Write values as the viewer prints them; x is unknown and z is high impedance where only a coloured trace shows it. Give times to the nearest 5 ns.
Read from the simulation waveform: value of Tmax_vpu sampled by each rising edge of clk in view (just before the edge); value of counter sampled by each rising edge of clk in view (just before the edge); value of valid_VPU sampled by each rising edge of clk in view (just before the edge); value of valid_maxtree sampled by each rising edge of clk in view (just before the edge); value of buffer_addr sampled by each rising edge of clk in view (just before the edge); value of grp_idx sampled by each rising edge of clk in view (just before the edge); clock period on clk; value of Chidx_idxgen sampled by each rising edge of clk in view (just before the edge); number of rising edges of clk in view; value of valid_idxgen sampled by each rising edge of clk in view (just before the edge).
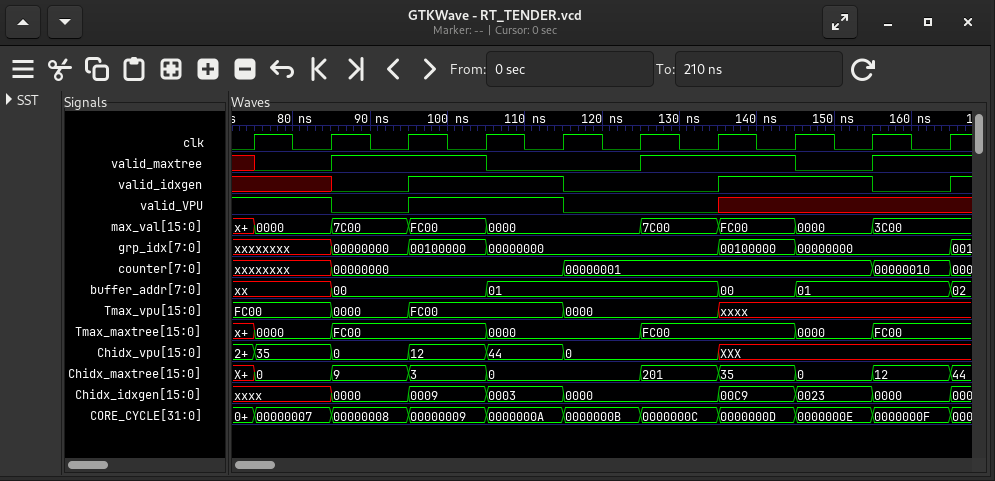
FC00, FC00, 0000, FC00, FC00, 0000, 0000, xxxx, xxxx, xxxx
xxxxxxxx, xxxxxxxx, 00000000, 00000000, 00000000, 00000001, 00000001, 00000001, 00000001, 00000010
1 1 0 1 1 0 0 x x x
x 0 1 1 0 0 1 1 0 1
xx, xx, 00, 00, 01, 01, 01, 00, 01, 01
xxxxxxxx, xxxxxxxx, 00000000, 00100000, 00000000, 00000000, 00000000, 00100000, 00000000, 00000000
10 ns
xxxx, xxxx, 0000, 0009, 0003, 0000, 0000, 00C9, 0023, 0000
10
x x 0 1 1 0 0 1 1 0
